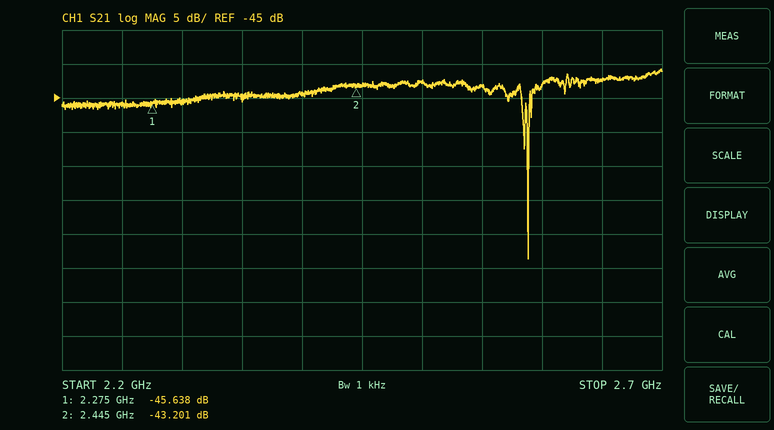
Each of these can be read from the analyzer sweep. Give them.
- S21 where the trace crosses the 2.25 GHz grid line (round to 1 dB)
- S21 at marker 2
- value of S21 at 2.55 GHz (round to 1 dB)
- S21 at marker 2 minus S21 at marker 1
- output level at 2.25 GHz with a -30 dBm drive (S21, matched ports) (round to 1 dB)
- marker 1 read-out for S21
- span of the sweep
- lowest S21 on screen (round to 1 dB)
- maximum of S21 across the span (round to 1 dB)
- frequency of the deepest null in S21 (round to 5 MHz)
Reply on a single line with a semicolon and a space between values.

-46 dB; -43.201 dB; -43 dB; 2.437 dB; -76 dBm; -45.638 dB; 500 MHz; -69 dB; -41 dB; 2.590 GHz
